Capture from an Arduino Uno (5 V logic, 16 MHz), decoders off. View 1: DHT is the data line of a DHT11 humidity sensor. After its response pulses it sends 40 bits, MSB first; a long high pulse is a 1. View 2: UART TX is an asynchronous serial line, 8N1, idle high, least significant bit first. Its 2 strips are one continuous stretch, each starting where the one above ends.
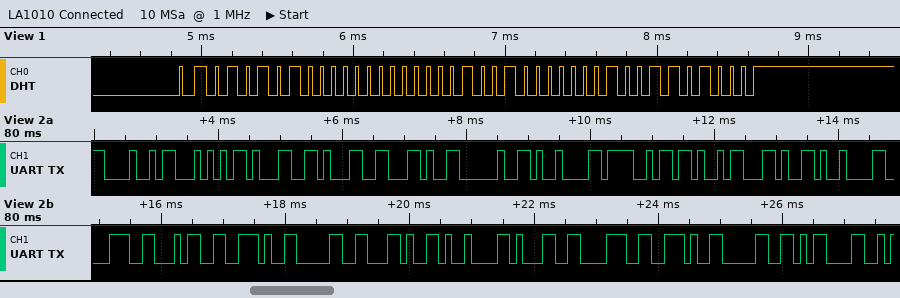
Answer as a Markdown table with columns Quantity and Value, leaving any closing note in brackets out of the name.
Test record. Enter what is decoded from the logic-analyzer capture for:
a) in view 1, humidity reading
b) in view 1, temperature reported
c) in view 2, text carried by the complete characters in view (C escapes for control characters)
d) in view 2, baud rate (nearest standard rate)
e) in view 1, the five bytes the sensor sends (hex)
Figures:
| Quantity | Value |
|---|---|
| in view 1, humidity reading | 84 % |
| in view 1, temperature reported | 18.2 °C |
| in view 2, text carried by the complete characters in view | "HT11, \tOK,\t84.0,\t18.0\r" |
| in view 2, baud rate | 9600 baud |
| in view 1, the five bytes the sensor sends | 54 00 12 02 68 |
